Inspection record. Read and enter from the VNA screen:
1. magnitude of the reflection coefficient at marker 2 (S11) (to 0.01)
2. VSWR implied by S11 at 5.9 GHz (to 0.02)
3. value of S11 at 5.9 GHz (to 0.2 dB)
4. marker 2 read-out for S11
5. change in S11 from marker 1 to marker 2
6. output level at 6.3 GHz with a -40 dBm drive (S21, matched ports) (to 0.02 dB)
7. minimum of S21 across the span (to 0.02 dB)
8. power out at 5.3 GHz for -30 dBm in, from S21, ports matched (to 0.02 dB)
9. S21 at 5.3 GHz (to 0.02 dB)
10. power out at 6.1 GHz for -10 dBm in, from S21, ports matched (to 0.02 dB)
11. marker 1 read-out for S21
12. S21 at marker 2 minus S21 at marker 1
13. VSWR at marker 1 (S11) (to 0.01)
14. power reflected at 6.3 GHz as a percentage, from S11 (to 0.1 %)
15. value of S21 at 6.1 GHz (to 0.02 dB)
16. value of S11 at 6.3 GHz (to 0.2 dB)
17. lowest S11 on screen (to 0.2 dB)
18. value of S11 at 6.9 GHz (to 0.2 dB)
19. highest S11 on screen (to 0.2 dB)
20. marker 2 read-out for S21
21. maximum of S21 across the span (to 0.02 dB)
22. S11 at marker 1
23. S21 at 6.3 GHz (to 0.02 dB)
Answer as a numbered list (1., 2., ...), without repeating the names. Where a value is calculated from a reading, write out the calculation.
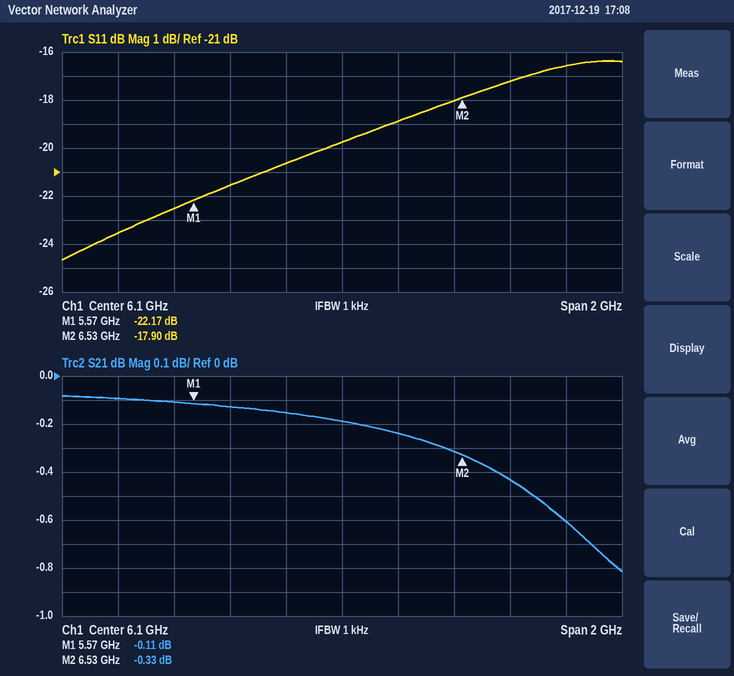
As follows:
1. 10^(-17.9/20) ≈ 0.13
2. |Γ| = 10^(-20.6/20) = 0.0933; VSWR = (1 + 0.0933)/(1 − 0.0933) ≈ 1.21, so 1.20 to the nearest 0.02
3. -20.6 dB
4. -17.90 dB
5. -17.9 − (-22.17) = 4.27 dB
6. -40 dBm + (-0.24 dB) = -40.24 dBm
7. -0.82 dB
8. -30 dBm + (-0.10 dB) = -30.10 dBm
9. -0.10 dB
10. -10 dBm + (-0.18 dB) = -10.18 dBm
11. -0.11 dB
12. -0.33 − (-0.11) = -0.22 dB
13. (1 + 0.0779)/(1 − 0.0779) ≈ 1.17
14. 10^(-18.8/10) ≈ 1.3 %
15. -0.18 dB
16. -18.8 dB
17. -24.6 dB
18. -16.6 dB
19. -16.4 dB
20. -0.33 dB
21. -0.08 dB
22. -22.17 dB
23. -0.24 dB
